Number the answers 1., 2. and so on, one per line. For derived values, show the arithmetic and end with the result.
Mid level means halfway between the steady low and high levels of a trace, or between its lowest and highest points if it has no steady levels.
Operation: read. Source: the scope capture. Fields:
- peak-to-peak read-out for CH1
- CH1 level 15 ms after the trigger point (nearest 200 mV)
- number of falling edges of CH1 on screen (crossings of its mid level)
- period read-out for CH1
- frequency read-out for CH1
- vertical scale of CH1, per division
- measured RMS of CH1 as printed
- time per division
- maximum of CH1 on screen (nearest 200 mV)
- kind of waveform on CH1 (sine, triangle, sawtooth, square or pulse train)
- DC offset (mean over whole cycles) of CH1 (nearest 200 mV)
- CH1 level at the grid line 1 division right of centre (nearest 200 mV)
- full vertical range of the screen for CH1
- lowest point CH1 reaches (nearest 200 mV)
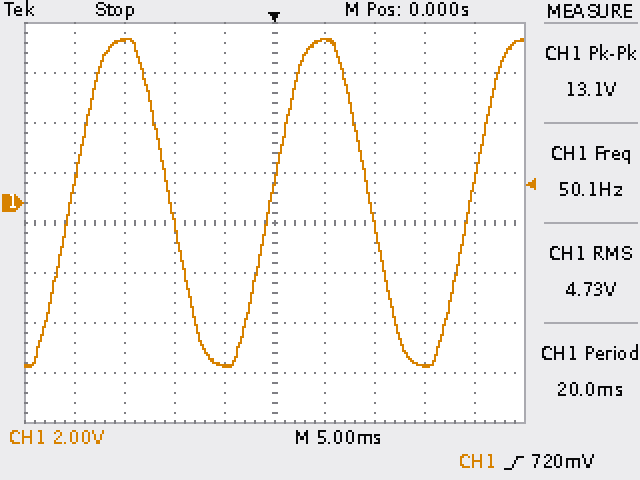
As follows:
1. 13.1 V
2. -6.6 V
3. 2
4. 20.0 ms
5. 50.1 Hz
6. 2 V
7. 4.73 V
8. 5 ms
9. 6.6 V
10. sine
11. (6.6 V + (-6.6 V)) / 2 ≈ 0.0 V
12. 6.6 V
13. 16 V
14. -6.6 V
